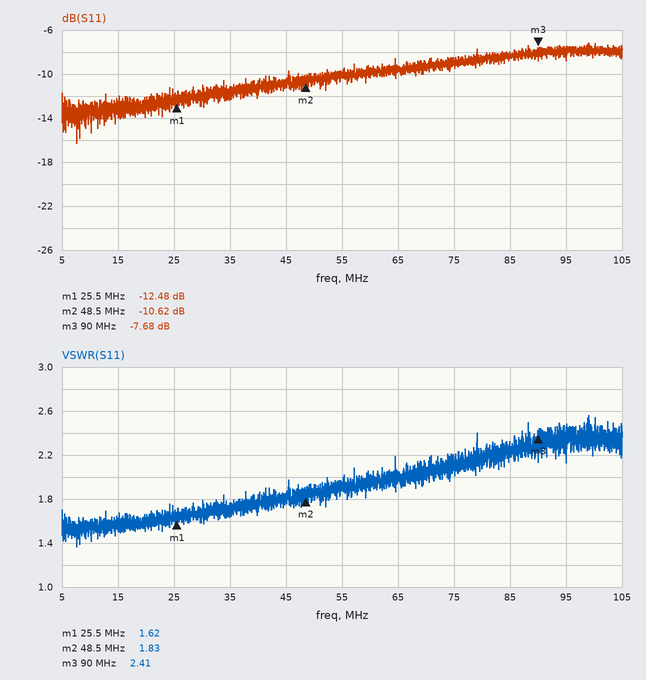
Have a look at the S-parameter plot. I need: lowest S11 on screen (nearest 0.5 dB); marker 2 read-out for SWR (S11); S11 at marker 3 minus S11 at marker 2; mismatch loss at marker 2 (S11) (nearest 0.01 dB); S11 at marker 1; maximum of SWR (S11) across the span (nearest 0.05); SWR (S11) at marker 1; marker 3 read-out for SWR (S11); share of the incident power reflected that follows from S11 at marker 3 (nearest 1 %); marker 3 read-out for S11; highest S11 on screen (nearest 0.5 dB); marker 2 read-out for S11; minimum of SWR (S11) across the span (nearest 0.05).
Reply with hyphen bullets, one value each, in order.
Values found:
- -16.5 dB
- 1.83
- 2.94 dB
- 0.39 dB
- -12.48 dB
- 2.55
- 1.62
- 2.41
- 17 %
- -7.68 dB
- -7.0 dB
- -10.62 dB
- 1.35
